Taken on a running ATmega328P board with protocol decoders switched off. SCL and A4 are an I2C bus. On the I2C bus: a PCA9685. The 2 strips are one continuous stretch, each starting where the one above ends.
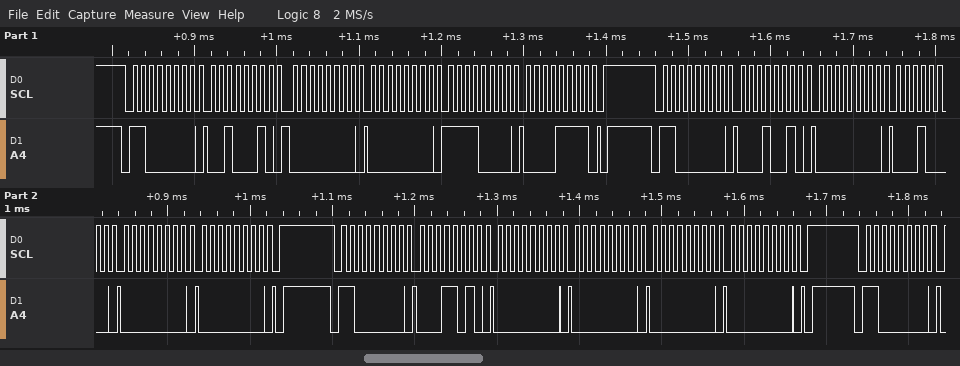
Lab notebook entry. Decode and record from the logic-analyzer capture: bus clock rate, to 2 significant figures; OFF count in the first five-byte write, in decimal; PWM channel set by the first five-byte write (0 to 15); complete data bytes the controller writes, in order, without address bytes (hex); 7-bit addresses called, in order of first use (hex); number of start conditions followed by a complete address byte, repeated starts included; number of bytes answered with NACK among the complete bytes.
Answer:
100 kHz
4080
7
22 00 00 F0 0F 12 00 10 00 00 1A 00 00 00 00
0x60
4
0
